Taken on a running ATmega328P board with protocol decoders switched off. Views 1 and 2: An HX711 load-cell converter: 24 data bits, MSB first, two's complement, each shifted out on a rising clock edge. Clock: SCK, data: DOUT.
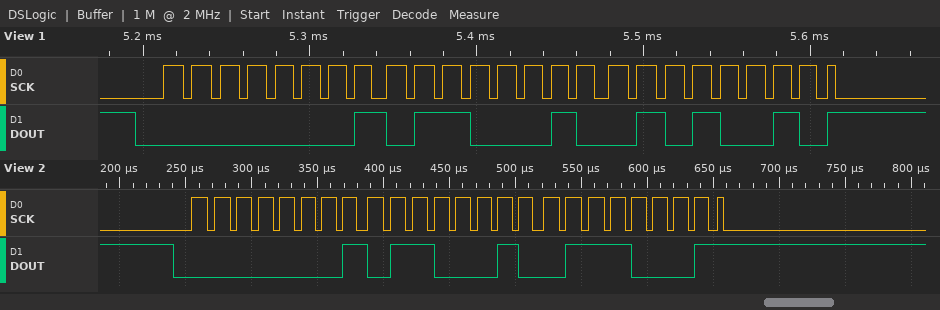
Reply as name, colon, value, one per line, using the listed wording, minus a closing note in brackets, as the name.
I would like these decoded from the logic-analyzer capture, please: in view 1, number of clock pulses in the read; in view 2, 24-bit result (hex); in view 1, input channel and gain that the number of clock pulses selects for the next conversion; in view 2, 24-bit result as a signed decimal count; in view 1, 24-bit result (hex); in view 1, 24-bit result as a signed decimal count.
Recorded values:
in view 1, number of clock pulses in the read: 25
in view 2, 24-bit result: 0x016271
in view 1, input channel and gain that the number of clock pulses selects for the next conversion: channel A, gain 128
in view 2, 24-bit result as a signed decimal count: 90737
in view 1, 24-bit result: 0x016252
in view 1, 24-bit result as a signed decimal count: 90706
